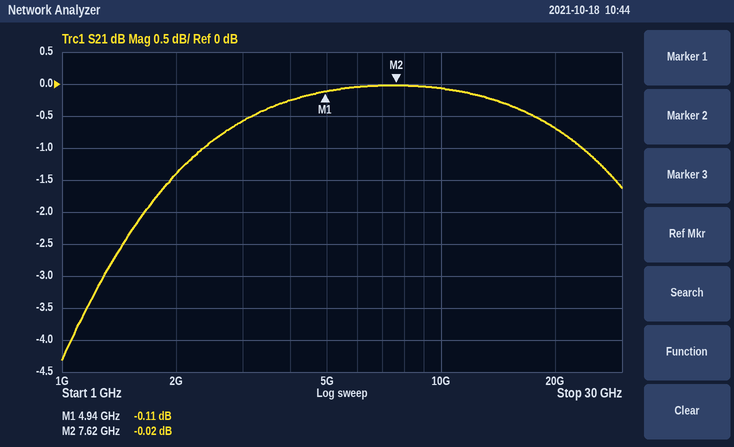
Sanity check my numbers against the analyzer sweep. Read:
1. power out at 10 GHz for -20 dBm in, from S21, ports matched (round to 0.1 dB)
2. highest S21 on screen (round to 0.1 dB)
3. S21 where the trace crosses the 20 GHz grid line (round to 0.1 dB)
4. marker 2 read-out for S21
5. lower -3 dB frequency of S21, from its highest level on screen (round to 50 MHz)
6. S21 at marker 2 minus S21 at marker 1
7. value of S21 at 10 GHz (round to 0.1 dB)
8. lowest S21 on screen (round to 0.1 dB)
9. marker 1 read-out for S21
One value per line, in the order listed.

-20.1 dBm
0.0 dB
-0.7 dB
-0.02 dB
1.30 GHz
0.09 dB
-0.1 dB
-4.3 dB
-0.11 dB
